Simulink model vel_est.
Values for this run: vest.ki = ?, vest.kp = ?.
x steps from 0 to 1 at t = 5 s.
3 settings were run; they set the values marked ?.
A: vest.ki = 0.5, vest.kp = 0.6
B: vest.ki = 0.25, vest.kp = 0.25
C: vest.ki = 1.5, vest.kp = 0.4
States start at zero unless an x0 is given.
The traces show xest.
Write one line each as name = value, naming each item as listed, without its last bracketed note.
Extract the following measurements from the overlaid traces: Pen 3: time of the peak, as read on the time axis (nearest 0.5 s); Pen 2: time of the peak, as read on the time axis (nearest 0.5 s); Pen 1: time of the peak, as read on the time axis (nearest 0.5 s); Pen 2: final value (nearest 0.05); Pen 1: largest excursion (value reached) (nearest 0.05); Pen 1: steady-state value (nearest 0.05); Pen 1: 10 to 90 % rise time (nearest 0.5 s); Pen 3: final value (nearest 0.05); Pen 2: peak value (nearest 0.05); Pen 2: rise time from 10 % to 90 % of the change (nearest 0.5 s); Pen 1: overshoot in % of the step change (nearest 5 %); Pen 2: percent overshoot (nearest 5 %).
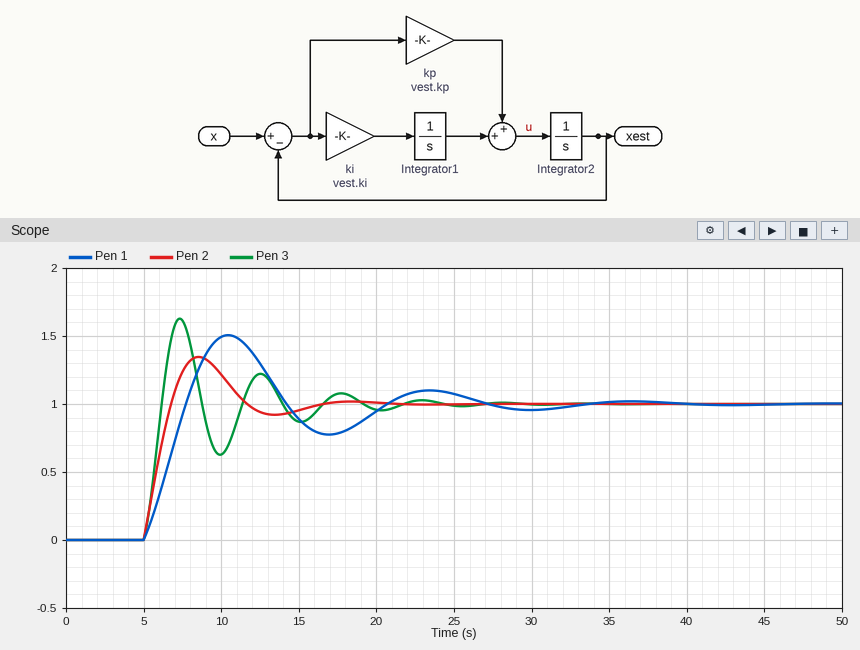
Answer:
Pen 3: time of the peak, as read on the time axis = 7.5 s
Pen 2: time of the peak, as read on the time axis = 8.5 s
Pen 1: time of the peak, as read on the time axis = 10.5 s
Pen 2: final value = 1.00
Pen 1: largest excursion (value reached) = 1.50
Pen 1: steady-state value = 1.00
Pen 1: 10 to 90 % rise time = 2.0 s
Pen 3: final value = 1.00
Pen 2: peak value = 1.35
Pen 2: rise time from 10 % to 90 % of the change = 1.5 s
Pen 1: overshoot in % of the step change = 50 %
Pen 2: percent overshoot = 35 %
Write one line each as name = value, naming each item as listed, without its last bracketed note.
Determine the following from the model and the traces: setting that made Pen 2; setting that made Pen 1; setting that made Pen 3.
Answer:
setting that made Pen 2 = A
setting that made Pen 1 = B
setting that made Pen 3 = C
